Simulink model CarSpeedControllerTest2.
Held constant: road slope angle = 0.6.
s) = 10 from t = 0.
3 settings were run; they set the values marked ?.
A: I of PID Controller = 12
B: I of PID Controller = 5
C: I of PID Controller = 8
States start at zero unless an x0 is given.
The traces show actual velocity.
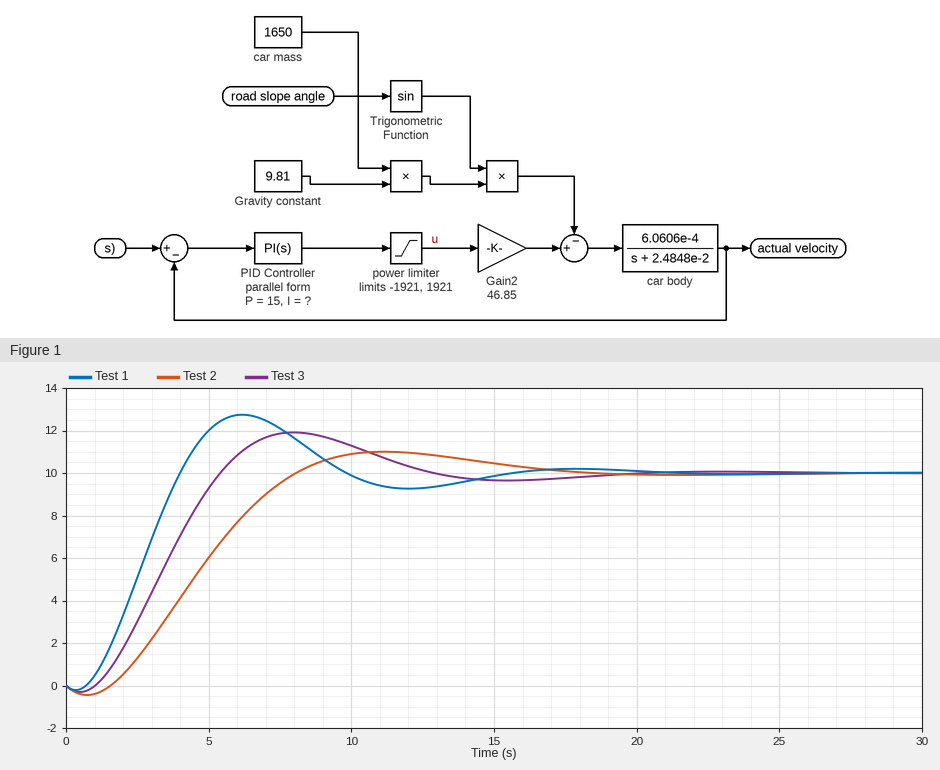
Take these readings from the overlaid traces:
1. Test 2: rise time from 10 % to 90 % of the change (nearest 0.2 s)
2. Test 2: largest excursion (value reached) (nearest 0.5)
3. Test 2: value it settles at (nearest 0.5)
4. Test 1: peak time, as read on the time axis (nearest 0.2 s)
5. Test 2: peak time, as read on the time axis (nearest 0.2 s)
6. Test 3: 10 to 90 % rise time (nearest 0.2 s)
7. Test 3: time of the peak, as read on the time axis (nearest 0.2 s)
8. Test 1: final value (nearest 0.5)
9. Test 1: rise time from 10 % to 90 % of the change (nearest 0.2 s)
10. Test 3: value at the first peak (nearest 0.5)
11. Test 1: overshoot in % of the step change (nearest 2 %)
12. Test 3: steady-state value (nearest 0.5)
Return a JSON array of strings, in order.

["4.6 s", "11.0", "10.0", "6.2 s", "11.2 s", "3.2 s", "8.0 s", "10.0", "2.4 s", "12.0", "28 %", "10.0"]
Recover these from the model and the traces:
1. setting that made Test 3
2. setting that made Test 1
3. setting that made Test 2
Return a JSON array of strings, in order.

["C", "A", "B"]
